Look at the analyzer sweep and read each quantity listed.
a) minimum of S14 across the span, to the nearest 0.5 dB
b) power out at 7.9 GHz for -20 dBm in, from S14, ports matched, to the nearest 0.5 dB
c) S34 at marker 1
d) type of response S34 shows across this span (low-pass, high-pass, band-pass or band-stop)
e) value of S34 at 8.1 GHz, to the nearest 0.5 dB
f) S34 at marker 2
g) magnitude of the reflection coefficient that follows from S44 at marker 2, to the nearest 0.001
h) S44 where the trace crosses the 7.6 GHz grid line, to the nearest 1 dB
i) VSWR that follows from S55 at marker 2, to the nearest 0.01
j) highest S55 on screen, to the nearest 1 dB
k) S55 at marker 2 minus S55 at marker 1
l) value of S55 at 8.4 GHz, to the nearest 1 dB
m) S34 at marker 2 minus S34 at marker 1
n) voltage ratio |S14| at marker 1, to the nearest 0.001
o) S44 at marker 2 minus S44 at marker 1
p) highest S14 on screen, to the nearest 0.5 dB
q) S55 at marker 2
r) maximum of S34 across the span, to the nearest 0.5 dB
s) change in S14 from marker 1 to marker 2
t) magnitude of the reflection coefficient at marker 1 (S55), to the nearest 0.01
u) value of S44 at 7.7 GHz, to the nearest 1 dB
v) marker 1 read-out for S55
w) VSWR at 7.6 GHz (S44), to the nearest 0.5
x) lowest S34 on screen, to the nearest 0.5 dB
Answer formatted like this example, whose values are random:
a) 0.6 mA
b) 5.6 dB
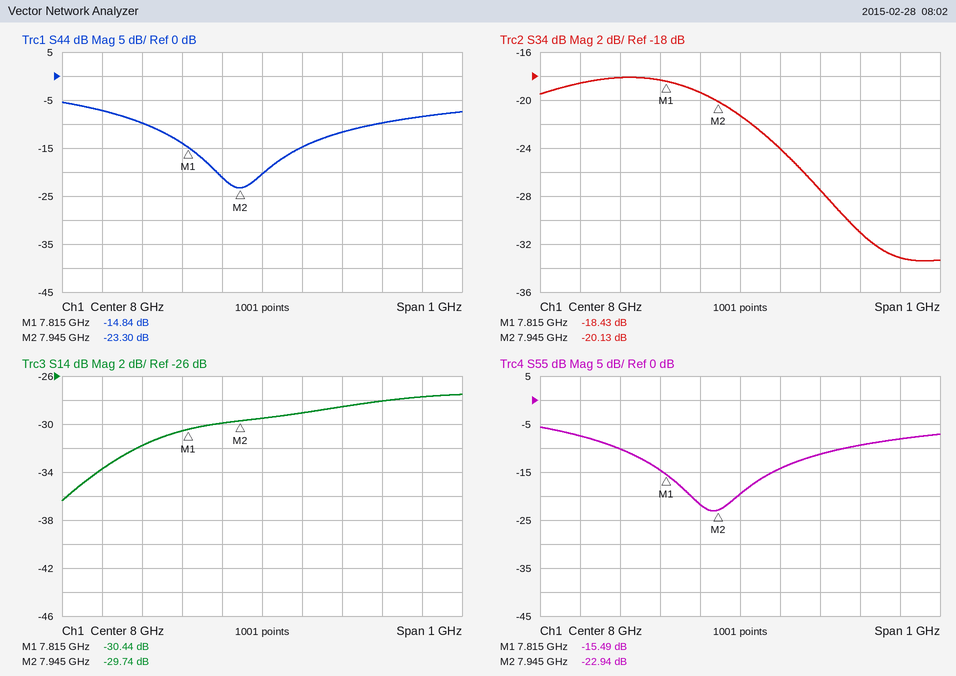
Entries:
a) -36.5 dB
b) -50.0 dBm
c) -18.43 dB
d) low-pass
e) -24.0 dB
f) -20.13 dB
g) 0.068
h) -7 dB
i) 1.15
j) -6 dB
k) -7.45 dB
l) -8 dB
m) -1.70 dB
n) 0.030
o) -8.46 dB
p) -27.5 dB
q) -22.94 dB
r) -18.0 dB
s) 0.70 dB
t) 0.17
u) -10 dB
v) -15.49 dB
w) 2.5
x) -33.5 dB
